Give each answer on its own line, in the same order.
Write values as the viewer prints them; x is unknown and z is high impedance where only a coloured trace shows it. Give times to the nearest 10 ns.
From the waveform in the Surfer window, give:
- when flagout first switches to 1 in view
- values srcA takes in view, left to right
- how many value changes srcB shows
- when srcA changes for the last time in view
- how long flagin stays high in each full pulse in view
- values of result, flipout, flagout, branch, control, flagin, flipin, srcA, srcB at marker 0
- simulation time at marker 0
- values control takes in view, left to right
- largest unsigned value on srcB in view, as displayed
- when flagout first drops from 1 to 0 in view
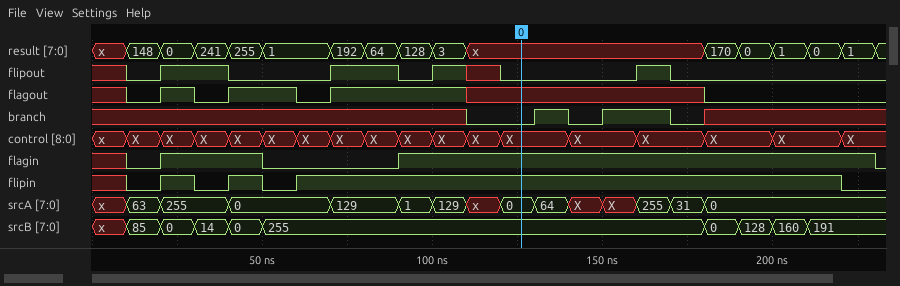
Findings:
20 ns
x, 63, 255, 0, 129, 1, 129, x, 0, 64, X, X, 255, 31, 0
9
180 ns
30 ns, 140 ns
result=x, flipout=0, flagout=x, branch=0, control=X, flagin=1, flipin=1, srcA=0, srcB=255
130 ns
x, X, X, X, X, X, X, X, X, X, X, X, X, X, X, X, X, X
255
30 ns
